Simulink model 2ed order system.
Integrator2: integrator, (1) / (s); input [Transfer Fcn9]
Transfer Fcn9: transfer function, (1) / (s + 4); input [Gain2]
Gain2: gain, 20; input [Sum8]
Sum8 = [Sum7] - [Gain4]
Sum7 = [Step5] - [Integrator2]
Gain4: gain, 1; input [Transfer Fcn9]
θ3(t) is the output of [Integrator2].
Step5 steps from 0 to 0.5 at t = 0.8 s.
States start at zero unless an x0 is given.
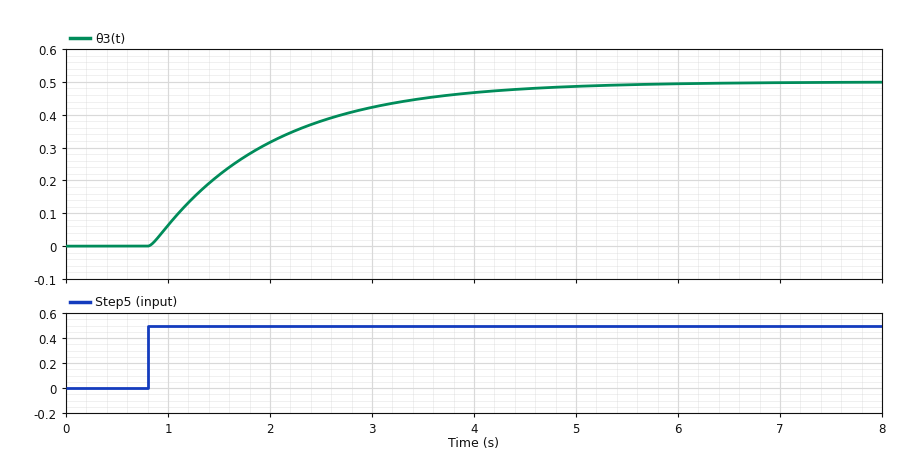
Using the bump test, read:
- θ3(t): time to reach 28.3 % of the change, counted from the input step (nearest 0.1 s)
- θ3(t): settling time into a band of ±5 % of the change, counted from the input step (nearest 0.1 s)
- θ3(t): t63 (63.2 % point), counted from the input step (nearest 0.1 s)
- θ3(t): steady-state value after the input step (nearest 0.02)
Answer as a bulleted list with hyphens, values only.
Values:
- 0.4 s
- 3.5 s
- 1.2 s
- 0.50
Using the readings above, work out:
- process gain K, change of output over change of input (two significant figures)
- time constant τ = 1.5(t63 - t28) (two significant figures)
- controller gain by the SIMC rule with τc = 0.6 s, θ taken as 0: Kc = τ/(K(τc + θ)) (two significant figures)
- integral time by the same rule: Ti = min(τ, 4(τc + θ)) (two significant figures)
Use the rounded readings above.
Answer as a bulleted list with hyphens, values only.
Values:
- 1.0
- 1.2 s
- 2.0
- 1.2 s
